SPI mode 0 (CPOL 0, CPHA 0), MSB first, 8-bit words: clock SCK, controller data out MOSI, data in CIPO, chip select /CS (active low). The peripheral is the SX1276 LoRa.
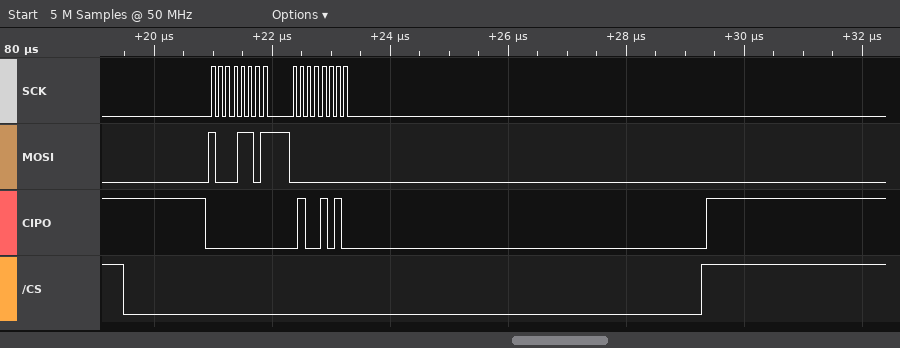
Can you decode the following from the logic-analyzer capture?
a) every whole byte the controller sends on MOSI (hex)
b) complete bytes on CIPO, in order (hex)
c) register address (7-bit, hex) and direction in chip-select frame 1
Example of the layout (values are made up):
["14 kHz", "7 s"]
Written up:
["8D 00", "00 4A", "0x0D write"]
